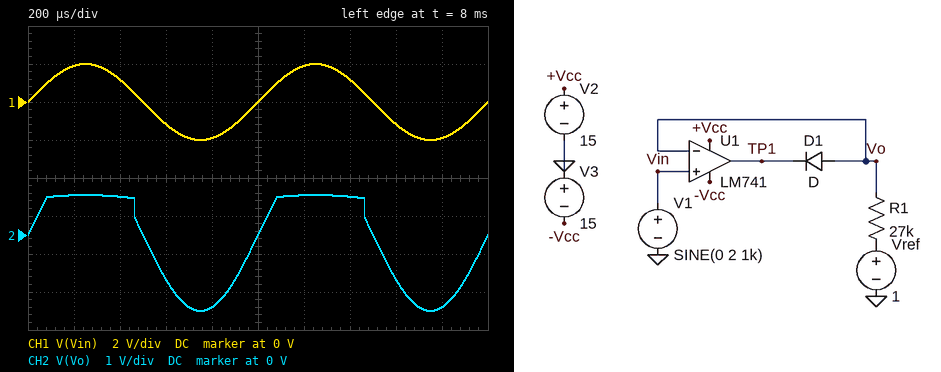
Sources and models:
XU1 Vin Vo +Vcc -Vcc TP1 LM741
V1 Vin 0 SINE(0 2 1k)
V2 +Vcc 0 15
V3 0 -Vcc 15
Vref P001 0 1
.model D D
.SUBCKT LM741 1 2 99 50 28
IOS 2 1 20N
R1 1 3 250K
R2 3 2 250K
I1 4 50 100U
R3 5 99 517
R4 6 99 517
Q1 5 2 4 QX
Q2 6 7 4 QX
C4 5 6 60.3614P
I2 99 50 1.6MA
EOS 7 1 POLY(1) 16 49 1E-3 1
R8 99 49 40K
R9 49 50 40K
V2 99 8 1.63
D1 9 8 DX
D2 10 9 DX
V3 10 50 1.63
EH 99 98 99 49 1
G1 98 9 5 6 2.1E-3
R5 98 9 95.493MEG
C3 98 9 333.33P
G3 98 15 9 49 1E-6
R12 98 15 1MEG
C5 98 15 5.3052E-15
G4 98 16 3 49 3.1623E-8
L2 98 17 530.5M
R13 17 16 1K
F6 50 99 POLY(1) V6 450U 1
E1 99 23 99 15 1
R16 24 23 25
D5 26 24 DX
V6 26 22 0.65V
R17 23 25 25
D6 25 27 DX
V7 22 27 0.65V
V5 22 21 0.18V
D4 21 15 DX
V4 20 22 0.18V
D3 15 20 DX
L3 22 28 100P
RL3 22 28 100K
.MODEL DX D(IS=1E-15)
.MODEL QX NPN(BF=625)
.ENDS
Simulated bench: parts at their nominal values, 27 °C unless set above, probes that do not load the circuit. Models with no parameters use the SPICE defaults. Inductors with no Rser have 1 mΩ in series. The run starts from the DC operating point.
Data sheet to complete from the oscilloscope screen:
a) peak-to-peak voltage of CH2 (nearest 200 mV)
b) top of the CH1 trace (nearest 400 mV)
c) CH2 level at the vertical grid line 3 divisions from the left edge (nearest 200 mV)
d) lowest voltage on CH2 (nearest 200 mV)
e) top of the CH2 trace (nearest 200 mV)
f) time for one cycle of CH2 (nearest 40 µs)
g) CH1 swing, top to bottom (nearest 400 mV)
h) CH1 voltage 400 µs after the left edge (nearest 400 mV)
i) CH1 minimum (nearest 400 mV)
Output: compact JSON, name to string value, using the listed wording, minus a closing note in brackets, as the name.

{"peak-to-peak voltage of CH2": "3.0 V", "top of the CH1 trace": "2.0 V", "CH2 level at the vertical grid line 3 divisions from the left edge": "-1.2 V", "lowest voltage on CH2": "-2.0 V", "top of the CH2 trace": "1.0 V", "time for one cycle of CH2": "1.00 ms", "CH1 swing, top to bottom": "4.0 V", "CH1 voltage 400 µs after the left edge": "1.2 V", "CH1 minimum": "-2.0 V"}
